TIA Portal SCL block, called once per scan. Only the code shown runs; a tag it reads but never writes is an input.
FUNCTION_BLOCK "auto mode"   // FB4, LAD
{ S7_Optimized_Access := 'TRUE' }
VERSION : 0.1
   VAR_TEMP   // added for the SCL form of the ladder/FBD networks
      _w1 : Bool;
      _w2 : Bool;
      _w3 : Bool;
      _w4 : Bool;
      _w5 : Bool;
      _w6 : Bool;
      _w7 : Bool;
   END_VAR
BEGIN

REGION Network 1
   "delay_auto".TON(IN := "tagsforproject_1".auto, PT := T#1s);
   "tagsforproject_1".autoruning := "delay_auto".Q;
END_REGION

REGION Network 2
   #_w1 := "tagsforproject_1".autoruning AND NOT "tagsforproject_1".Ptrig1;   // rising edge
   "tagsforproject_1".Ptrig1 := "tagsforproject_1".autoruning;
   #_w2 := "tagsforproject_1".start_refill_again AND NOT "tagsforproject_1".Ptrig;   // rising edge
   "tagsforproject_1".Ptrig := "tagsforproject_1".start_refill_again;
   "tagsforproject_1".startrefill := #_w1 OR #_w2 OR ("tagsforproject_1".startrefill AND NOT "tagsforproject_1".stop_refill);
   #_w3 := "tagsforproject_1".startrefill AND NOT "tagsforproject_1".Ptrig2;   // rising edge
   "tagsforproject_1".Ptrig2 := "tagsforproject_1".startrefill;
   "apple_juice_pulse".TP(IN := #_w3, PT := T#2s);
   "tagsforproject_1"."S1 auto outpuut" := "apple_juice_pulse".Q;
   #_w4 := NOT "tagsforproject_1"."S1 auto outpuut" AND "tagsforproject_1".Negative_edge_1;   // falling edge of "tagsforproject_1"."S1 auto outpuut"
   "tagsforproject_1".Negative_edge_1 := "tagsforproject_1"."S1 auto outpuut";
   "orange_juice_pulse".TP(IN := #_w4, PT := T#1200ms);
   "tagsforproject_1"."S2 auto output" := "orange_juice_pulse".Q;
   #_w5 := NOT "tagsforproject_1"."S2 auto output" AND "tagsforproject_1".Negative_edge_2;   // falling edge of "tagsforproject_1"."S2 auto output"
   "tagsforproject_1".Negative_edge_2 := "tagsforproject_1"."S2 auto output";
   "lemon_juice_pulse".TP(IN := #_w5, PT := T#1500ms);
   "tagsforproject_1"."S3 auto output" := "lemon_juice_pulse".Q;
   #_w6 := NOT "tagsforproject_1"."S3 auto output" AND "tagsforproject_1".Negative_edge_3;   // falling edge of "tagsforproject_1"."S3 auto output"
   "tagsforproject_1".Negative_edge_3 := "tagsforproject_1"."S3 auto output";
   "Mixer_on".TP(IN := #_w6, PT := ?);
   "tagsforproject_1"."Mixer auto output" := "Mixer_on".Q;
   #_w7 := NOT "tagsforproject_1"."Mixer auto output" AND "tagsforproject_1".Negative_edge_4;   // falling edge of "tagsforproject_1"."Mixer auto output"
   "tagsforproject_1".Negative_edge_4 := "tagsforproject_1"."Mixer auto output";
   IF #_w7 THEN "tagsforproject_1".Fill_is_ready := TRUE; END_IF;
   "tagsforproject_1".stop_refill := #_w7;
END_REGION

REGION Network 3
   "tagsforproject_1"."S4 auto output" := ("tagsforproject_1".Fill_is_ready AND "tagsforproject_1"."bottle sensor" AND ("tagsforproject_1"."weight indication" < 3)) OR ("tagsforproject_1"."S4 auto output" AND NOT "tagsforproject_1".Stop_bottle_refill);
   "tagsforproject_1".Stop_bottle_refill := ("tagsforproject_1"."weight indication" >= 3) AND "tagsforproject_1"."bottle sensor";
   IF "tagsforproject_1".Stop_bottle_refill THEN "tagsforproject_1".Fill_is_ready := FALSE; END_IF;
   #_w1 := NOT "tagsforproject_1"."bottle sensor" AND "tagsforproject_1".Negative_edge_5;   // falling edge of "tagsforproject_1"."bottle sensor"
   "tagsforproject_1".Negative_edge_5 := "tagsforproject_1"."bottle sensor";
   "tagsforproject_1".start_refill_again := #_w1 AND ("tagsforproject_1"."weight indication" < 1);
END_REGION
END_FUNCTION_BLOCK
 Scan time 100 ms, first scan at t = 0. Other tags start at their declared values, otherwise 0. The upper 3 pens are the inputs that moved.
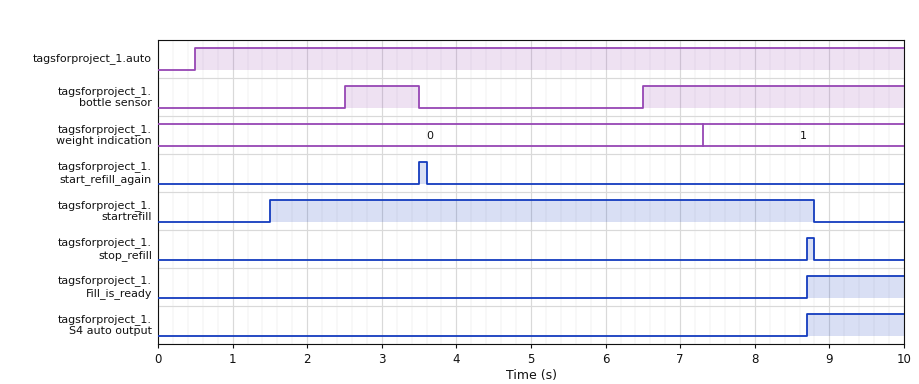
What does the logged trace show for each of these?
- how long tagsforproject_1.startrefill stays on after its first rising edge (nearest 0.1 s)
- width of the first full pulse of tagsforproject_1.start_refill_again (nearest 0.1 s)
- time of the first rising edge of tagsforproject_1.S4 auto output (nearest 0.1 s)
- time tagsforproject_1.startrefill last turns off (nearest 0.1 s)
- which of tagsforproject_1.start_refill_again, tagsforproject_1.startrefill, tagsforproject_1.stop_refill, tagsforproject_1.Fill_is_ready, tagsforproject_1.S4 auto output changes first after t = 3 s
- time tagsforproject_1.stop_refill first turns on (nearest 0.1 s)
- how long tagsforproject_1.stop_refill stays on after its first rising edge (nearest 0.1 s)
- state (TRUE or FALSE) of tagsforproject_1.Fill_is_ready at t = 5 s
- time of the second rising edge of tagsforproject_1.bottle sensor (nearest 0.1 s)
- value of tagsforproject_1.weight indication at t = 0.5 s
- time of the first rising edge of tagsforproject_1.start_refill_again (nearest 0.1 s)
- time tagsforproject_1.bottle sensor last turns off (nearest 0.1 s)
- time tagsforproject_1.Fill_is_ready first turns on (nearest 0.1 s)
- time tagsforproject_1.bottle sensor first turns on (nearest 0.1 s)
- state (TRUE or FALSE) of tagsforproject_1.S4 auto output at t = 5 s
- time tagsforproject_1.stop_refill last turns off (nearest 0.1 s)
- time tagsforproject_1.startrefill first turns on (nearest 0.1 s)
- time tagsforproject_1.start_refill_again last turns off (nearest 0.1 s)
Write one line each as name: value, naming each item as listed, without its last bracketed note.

how long tagsforproject_1.startrefill stays on after its first rising edge: 7.3 s
width of the first full pulse of tagsforproject_1.start_refill_again: 0.1 s
time of the first rising edge of tagsforproject_1.S4 auto output: 8.7 s
time tagsforproject_1.startrefill last turns off: 8.8 s
which of tagsforproject_1.start_refill_again, tagsforproject_1.startrefill, tagsforproject_1.stop_refill, tagsforproject_1.Fill_is_ready, tagsforproject_1.S4 auto output changes first after t = 3 s: tagsforproject_1.start_refill_again
time tagsforproject_1.stop_refill first turns on: 8.7 s
how long tagsforproject_1.stop_refill stays on after its first rising edge: 0.1 s
state (TRUE or FALSE) of tagsforproject_1.Fill_is_ready at t = 5 s: FALSE
time of the second rising edge of tagsforproject_1.bottle sensor: 6.5 s
value of tagsforproject_1.weight indication at t = 0.5 s: 0
time of the first rising edge of tagsforproject_1.start_refill_again: 3.5 s
time tagsforproject_1.bottle sensor last turns off: 3.5 s
time tagsforproject_1.Fill_is_ready first turns on: 8.7 s
time tagsforproject_1.bottle sensor first turns on: 2.5 s
state (TRUE or FALSE) of tagsforproject_1.S4 auto output at t = 5 s: FALSE
time tagsforproject_1.stop_refill last turns off: 8.8 s
time tagsforproject_1.startrefill first turns on: 1.5 s
time tagsforproject_1.start_refill_again last turns off: 3.6 s
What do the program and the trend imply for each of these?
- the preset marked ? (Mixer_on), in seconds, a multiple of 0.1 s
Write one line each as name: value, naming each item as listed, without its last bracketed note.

the preset marked ? (Mixer_on), in seconds, a multiple of 0.1 s: 2.5 s
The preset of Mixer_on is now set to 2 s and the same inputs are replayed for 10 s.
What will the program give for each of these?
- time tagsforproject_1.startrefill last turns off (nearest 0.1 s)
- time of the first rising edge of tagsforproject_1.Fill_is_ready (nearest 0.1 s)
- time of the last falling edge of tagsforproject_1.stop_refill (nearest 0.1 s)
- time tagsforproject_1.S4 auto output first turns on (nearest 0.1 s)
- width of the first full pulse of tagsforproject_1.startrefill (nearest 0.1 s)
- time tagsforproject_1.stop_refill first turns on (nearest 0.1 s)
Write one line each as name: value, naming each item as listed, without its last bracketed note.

time tagsforproject_1.startrefill last turns off: 8.3 s
time of the first rising edge of tagsforproject_1.Fill_is_ready: 8.2 s
time of the last falling edge of tagsforproject_1.stop_refill: 8.3 s
time tagsforproject_1.S4 auto output first turns on: 8.2 s
width of the first full pulse of tagsforproject_1.startrefill: 6.8 s
time tagsforproject_1.stop_refill first turns on: 8.2 s
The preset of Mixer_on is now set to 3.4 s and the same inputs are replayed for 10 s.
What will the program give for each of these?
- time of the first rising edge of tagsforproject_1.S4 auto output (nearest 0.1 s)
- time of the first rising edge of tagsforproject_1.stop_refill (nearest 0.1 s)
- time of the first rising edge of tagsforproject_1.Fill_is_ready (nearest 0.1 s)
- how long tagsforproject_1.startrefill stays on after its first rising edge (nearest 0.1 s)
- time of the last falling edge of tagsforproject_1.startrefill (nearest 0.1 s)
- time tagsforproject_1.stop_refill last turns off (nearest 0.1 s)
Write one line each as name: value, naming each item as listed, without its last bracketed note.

time of the first rising edge of tagsforproject_1.S4 auto output: 9.6 s
time of the first rising edge of tagsforproject_1.stop_refill: 9.6 s
time of the first rising edge of tagsforproject_1.Fill_is_ready: 9.6 s
how long tagsforproject_1.startrefill stays on after its first rising edge: 8.2 s
time of the last falling edge of tagsforproject_1.startrefill: 9.7 s
time tagsforproject_1.stop_refill last turns off: 9.7 s
